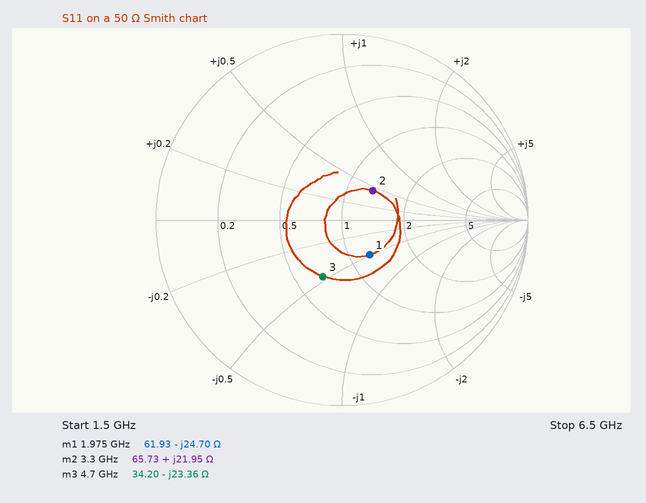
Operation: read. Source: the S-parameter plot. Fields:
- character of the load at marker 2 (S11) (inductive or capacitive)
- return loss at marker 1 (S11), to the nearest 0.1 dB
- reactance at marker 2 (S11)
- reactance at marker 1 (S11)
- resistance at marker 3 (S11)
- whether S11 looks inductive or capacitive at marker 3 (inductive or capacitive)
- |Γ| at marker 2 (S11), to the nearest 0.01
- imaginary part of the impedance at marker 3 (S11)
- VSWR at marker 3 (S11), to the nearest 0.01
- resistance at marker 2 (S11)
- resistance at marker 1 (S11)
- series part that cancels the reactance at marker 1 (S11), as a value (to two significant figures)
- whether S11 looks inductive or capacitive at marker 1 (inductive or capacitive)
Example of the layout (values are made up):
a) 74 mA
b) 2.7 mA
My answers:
a) inductive
b) 12.4 dB
c) +21.95 Ω
d) -24.70 Ω
e) 34.20 Ω
f) capacitive
g) 0.23
h) -23.36 Ω
i) 1.95
j) 65.73 Ω
k) 61.93 Ω
l) 2.0 nH
m) capacitive
